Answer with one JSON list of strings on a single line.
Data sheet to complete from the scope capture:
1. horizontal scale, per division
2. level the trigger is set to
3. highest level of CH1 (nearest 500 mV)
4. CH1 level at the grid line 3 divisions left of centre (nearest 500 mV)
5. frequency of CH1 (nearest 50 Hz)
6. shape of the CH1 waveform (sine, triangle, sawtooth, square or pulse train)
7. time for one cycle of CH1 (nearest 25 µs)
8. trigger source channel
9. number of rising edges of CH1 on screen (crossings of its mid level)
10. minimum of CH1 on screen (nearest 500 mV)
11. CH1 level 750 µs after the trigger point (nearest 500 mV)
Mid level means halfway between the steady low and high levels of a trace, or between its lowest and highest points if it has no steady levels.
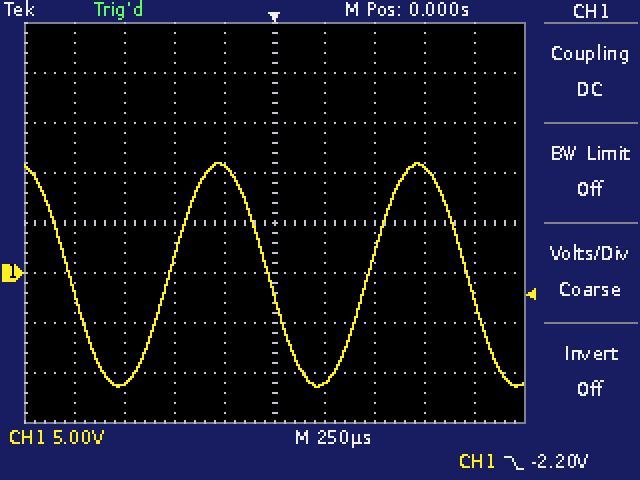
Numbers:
["250 µs", "-2.20 V", "11.0 V", "-11.0 V", "1.00 kHz", "sine", "1.000 ms", "CH1", "2", "-11.5 V", "10.5 V"]
